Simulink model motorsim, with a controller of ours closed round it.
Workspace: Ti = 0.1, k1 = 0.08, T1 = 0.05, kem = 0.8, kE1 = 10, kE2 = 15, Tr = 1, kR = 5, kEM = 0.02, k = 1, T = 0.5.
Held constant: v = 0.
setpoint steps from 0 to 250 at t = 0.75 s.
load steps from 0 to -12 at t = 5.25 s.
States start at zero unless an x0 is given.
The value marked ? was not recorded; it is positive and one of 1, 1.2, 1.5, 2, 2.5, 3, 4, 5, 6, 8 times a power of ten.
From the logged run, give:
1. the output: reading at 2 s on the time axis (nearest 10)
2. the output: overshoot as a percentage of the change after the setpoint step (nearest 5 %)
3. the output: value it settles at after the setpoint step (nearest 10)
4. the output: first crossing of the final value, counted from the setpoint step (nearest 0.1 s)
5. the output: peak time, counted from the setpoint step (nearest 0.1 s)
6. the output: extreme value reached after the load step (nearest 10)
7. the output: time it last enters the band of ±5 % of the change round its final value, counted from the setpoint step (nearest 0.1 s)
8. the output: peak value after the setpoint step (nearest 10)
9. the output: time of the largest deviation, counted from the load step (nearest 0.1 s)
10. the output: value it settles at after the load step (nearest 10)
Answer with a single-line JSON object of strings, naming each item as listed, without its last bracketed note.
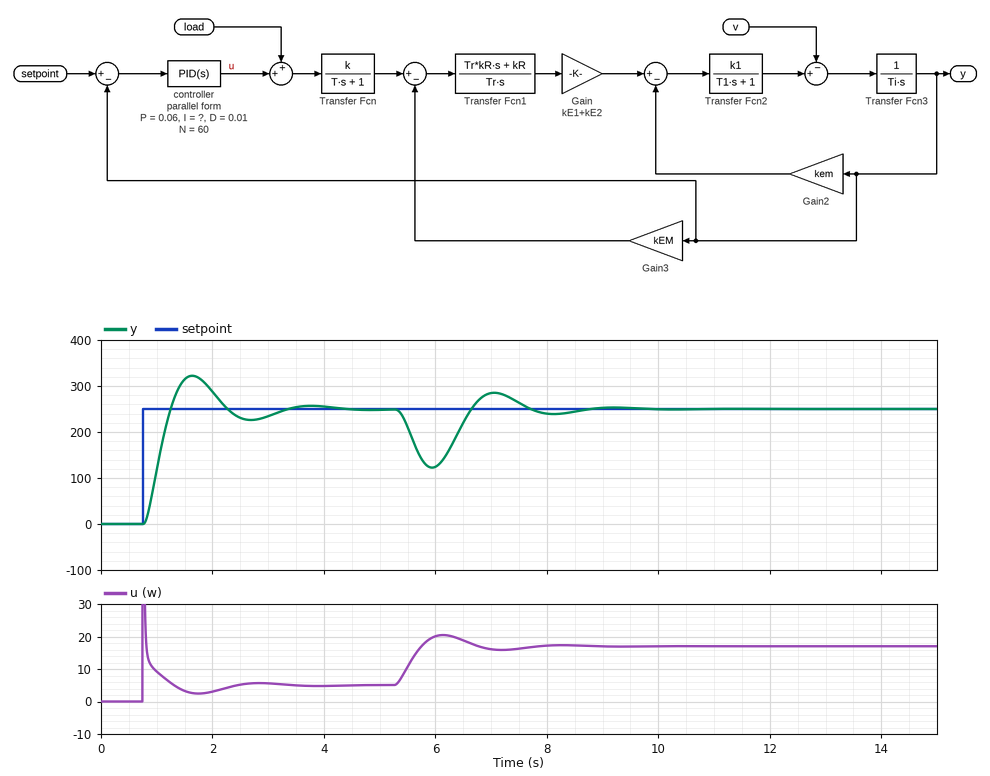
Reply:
{"the output: reading at 2 s on the time axis": "290", "the output: overshoot as a percentage of the change after the setpoint step": "30 %", "the output: value it settles at after the setpoint step": "250", "the output: first crossing of the final value, counted from the setpoint step": "0.5 s", "the output: peak time, counted from the setpoint step": "0.9 s", "the output: extreme value reached after the load step": "120", "the output: time it last enters the band of ±5 % of the change round its final value, counted from the setpoint step": "2.3 s", "the output: peak value after the setpoint step": "320", "the output: time of the largest deviation, counted from the load step": "0.7 s", "the output: value it settles at after the load step": "250"}
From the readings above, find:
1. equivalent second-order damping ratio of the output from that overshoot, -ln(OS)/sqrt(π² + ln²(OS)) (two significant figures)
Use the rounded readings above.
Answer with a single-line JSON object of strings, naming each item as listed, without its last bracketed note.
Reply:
{"equivalent second-order damping ratio of the output from that overshoot, -ln(OS)/sqrt(π² + ln²(OS))": "0.36"}
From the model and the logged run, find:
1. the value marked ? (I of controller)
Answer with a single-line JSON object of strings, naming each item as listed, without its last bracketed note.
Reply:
{"the value marked ?": "0.15"}
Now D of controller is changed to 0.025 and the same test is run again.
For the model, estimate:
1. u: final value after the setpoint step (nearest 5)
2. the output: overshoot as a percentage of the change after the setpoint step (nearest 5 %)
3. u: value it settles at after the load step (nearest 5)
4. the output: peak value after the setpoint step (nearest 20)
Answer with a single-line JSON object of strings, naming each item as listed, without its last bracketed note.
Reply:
{"u: final value after the setpoint step": "5", "the output: overshoot as a percentage of the change after the setpoint step": "10 %", "u: value it settles at after the load step": "15", "the output: peak value after the setpoint step": "280"}
